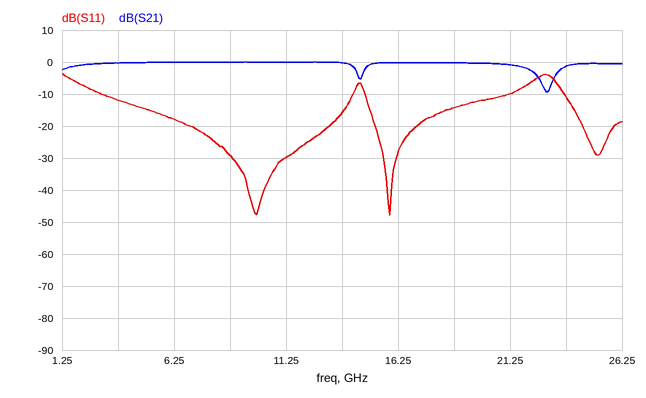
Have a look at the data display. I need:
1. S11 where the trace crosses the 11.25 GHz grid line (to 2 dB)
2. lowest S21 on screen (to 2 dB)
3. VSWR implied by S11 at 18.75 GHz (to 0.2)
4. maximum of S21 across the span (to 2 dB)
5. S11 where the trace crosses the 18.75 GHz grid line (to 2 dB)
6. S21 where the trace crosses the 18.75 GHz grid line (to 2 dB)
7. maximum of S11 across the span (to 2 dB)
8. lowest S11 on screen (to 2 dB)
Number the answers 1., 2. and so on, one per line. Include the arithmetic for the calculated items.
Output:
1. -30 dB
2. -10 dB
3. |Γ| = 10^(-14/20) = 0.1995; VSWR = (1 + 0.1995)/(1 − 0.1995) ≈ 1.50, so 1.4 to the nearest 0.2
4. 0 dB
5. -14 dB
6. 0 dB
7. -4 dB
8. -48 dB
